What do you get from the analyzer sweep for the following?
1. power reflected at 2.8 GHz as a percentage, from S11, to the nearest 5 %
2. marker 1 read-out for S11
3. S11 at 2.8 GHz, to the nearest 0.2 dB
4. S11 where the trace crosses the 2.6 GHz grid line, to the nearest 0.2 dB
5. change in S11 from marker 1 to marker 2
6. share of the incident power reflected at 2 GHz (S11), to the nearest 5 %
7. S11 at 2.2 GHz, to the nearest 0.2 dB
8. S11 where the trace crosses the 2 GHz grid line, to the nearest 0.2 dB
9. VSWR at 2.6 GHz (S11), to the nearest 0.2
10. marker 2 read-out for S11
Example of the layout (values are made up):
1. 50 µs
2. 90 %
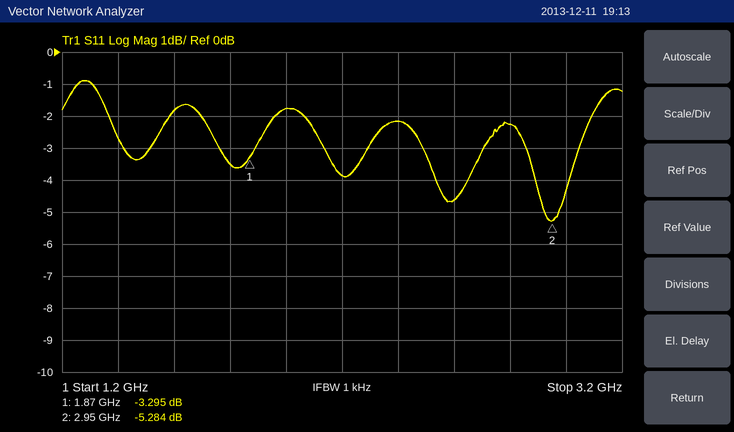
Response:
1. 60 %
2. -3.295 dB
3. -2.2 dB
4. -4.6 dB
5. -1.989 dB
6. 65 %
7. -3.8 dB
8. -1.8 dB
9. 3.8
10. -5.284 dB
